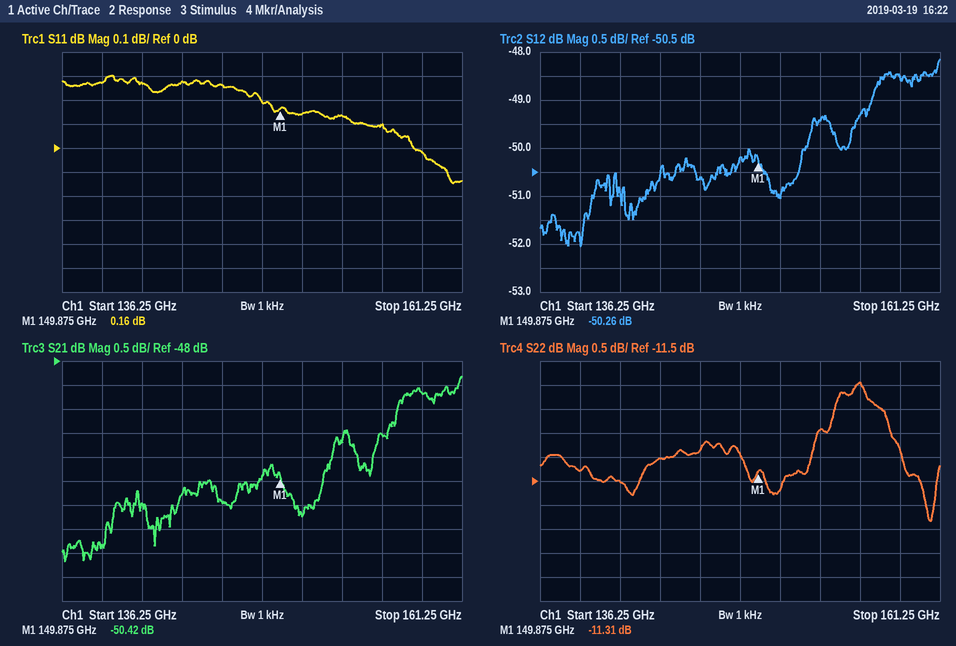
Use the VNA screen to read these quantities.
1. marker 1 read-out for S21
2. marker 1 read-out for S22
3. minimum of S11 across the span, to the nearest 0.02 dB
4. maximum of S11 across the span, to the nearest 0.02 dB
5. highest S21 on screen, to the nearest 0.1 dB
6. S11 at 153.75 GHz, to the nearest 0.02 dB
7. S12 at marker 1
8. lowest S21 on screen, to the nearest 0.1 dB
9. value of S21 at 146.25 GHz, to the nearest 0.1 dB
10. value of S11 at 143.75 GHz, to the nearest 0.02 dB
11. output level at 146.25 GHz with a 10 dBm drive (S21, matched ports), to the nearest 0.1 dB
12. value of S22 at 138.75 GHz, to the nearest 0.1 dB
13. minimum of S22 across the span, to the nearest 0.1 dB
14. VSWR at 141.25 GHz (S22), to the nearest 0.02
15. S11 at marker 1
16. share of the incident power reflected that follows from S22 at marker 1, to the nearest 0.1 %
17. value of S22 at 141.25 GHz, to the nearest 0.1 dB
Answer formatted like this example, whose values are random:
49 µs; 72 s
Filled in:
-50.42 dB; -11.31 dB; -0.14 dB; 0.30 dB; -48.3 dB; 0.14 dB; -50.26 dB; -52.2 dB; -50.9 dB; 0.28 dB; -40.9 dBm; -11.3 dB; -12.3 dB; 1.72; 0.16 dB; 7.4 %; -11.5 dB
